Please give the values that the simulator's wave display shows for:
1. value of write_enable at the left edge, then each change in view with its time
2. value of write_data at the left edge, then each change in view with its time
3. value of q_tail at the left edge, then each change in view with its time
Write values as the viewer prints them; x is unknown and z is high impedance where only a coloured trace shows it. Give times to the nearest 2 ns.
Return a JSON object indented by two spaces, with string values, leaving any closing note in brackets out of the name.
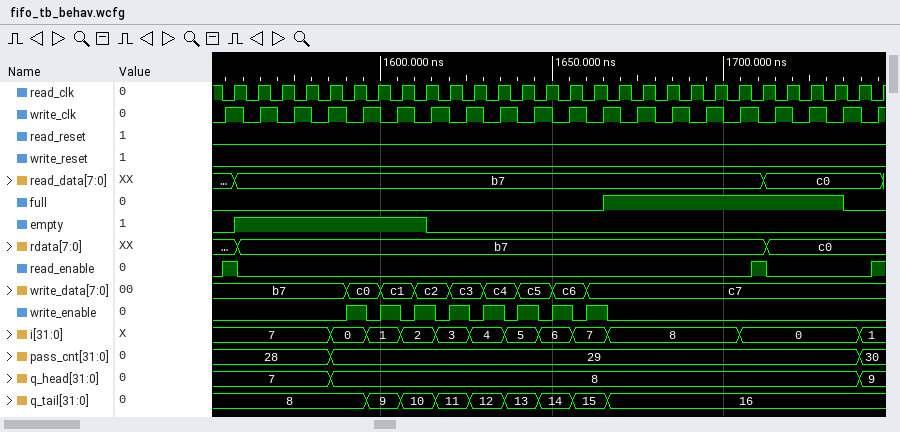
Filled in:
{
  "value of write_enable at the left edge, then each change in view with its time": "0, 1 at 1590 ns, 0 at 1596 ns, 1 at 1600 ns, 0 at 1606 ns, 1 at 1610 ns, 0 at 1616 ns, 1 at 1620 ns, 0 at 1626 ns, 1 at 1630 ns, 0 at 1636 ns, 1 at 1640 ns, 0 at 1646 ns, 1 at 1650 ns, 0 at 1656 ns, 1 at 1660 ns, 0 at 1666 ns",
  "value of write_data at the left edge, then each change in view with its time": "b7, c0 at 1590 ns, c1 at 1600 ns, c2 at 1610 ns, c3 at 1620 ns, c4 at 1630 ns, c5 at 1640 ns, c6 at 1650 ns, c7 at 1660 ns",
  "value of q_tail at the left edge, then each change in view with its time": "8, 9 at 1596 ns, 10 at 1606 ns, 11 at 1616 ns, 12 at 1626 ns, 13 at 1636 ns, 14 at 1646 ns, 15 at 1656 ns, 16 at 1666 ns"
}
